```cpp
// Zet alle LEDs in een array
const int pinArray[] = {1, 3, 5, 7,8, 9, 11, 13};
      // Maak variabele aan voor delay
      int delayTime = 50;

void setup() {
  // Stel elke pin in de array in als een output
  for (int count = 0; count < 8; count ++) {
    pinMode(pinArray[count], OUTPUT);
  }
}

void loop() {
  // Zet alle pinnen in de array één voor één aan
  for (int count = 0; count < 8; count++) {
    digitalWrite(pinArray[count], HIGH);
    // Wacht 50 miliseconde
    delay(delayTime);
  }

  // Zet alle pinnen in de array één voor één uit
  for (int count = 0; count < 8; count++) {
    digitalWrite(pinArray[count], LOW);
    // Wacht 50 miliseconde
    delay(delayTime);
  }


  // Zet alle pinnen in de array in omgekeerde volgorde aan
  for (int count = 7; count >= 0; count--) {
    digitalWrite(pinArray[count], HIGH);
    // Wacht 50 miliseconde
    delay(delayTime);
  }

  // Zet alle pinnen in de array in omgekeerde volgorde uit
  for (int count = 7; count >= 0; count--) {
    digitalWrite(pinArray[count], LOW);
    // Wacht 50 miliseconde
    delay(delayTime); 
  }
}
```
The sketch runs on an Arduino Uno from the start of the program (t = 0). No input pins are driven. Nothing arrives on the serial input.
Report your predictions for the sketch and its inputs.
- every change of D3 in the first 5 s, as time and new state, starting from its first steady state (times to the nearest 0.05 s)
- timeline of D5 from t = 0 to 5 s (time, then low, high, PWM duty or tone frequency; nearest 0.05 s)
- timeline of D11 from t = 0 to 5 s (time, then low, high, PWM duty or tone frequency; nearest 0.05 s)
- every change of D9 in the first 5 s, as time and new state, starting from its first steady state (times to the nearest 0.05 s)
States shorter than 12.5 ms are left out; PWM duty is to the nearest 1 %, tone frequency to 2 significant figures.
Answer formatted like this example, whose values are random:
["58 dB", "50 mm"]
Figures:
["0 s low; 0.05 s high; 0.45 s low; 1.1 s high; 1.5 s low; 1.65 s high; 2.05 s low; 2.7 s high; 3.1 s low; 3.25 s high; 3.65 s low; 4.3 s high; 4.7 s low; 4.85 s high", "0 s low; 0.1 s high; 0.5 s low; 1.05 s high; 1.45 s low; 1.7 s high; 2.1 s low; 2.65 s high; 3.05 s low; 3.3 s high; 3.7 s low; 4.25 s high; 4.65 s low; 4.9 s high", "0 s low; 0.3 s high; 0.7 s low; 0.85 s high; 1.25 s low; 1.9 s high; 2.3 s low; 2.45 s high; 2.85 s low; 3.5 s high; 3.9 s low; 4.05 s high; 4.45 s low", "0 s low; 0.25 s high; 0.65 s low; 0.9 s high; 1.3 s low; 1.85 s high; 2.25 s low; 2.5 s high; 2.9 s low; 3.45 s high; 3.85 s low; 4.1 s high; 4.5 s low"]
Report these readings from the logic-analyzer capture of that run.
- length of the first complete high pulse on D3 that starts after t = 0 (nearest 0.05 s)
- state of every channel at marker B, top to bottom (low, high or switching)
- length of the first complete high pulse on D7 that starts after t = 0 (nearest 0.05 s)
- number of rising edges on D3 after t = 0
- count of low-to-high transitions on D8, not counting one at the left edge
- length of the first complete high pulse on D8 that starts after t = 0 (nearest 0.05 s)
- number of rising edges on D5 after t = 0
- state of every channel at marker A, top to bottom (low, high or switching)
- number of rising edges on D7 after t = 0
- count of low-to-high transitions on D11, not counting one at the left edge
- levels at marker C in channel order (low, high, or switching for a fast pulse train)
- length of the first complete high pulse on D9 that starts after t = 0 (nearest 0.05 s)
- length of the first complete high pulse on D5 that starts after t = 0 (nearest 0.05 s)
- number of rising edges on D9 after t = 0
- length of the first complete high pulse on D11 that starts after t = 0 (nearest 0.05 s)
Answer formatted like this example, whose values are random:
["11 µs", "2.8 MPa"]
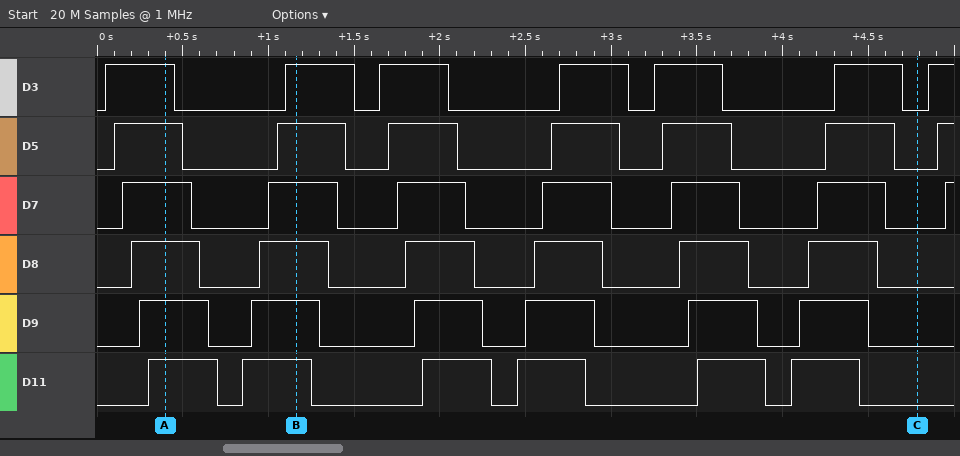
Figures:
["0.40 s", "D3 high, D5 high, D7 high, D8 high, D9 high, D11 high", "0.40 s", "7", "6", "0.40 s", "7", "D3 high, D5 high, D7 high, D8 high, D9 high, D11 high", "7", "6", "D3 low, D5 low, D7 low, D8 low, D9 low, D11 low", "0.40 s", "0.40 s", "6", "0.40 s"]
